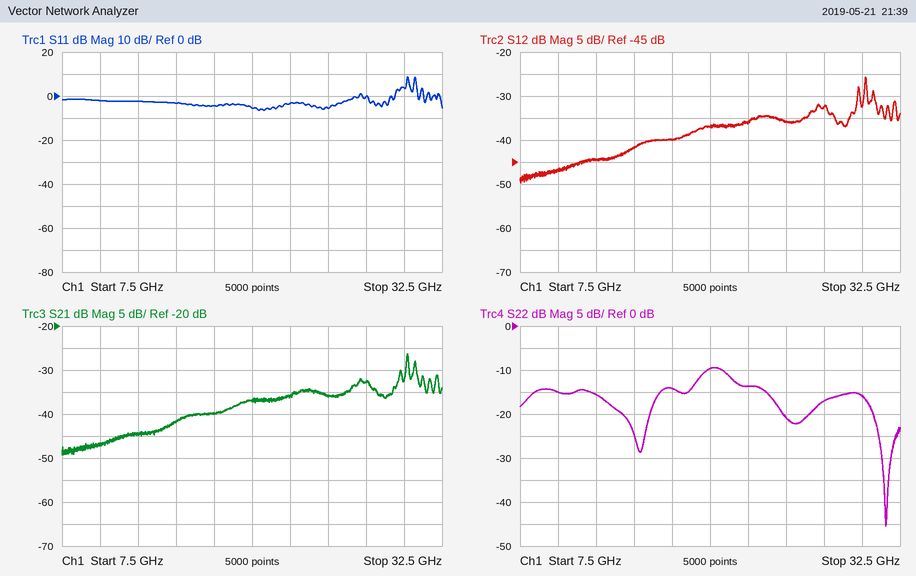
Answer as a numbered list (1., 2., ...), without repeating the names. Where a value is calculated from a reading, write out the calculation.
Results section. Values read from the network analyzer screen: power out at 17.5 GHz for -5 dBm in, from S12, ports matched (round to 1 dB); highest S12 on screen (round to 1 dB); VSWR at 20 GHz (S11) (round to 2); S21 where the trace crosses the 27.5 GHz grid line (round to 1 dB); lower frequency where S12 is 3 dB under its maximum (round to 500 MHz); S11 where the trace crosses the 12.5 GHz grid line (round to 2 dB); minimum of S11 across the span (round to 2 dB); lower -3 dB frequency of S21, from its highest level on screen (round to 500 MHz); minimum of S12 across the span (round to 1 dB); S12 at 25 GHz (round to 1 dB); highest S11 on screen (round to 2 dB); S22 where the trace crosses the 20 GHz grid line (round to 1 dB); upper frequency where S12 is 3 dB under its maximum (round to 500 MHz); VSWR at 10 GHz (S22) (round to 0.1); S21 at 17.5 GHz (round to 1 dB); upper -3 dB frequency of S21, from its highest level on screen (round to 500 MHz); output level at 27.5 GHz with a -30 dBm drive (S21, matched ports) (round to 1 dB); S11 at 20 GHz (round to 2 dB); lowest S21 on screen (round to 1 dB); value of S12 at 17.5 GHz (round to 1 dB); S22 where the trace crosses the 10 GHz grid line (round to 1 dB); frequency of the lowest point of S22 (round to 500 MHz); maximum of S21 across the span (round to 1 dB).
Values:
1. -5 dBm + (-40 dB) = -45 dBm
2. -26 dB
3. |Γ| = 10^(-6/20) = 0.5012; VSWR = (1 + 0.5012)/(1 − 0.5012) ≈ 3.01, so 4 to the nearest 2
4. -33 dB
5. 30.0 GHz
6. -2 dB
7. -6 dB
8. 30.0 GHz
9. -50 dB
10. -36 dB
11. 8 dB
12. -10 dB
13. 30.5 GHz
14. |Γ| = 10^(-15/20) = 0.1778; VSWR = (1 + 0.1778)/(1 − 0.1778) ≈ 1.4
15. -40 dB
16. 30.5 GHz
17. -30 dBm + (-33 dB) = -63 dBm
18. -6 dB
19. -49 dB
20. -40 dB
21. -15 dB
22. 31.5 GHz
23. -26 dB
